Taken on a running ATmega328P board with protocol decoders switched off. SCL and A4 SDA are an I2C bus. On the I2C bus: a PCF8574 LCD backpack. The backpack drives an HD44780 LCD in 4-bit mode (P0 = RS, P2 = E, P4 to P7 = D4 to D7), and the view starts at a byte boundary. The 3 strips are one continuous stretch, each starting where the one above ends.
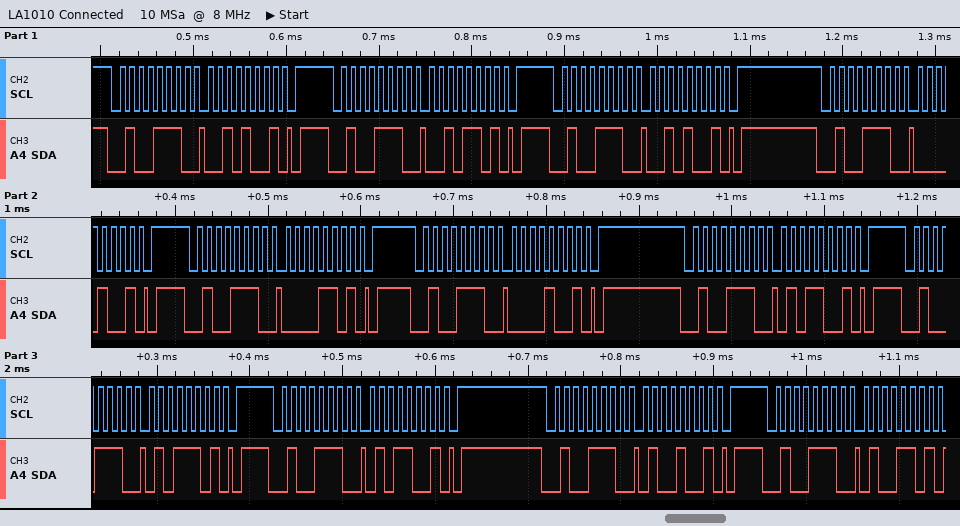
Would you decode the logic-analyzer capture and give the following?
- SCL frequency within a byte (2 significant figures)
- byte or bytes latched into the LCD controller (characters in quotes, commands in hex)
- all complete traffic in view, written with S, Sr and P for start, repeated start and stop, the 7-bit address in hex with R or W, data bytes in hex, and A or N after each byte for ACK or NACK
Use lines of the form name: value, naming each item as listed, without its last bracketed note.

SCL frequency within a byte: 100 kHz
byte or bytes latched into the LCD controller: ' '
all complete traffic in view, written with S, Sr and P for start, repeated start and stop, the 7-bit address in hex with R or W, data bytes in hex, and A or N after each byte for ACK or NACK: S 27W A 29 A P S 27W A 2D A P S 27W A 29 A P S 27W A 09 A P S 27W A 0D A P S 27W A 09 A P S 27W A 59 A P S 27W A 5D A P S 27W A 59 A P S 27W A 49 A P S 27W A 4D A
